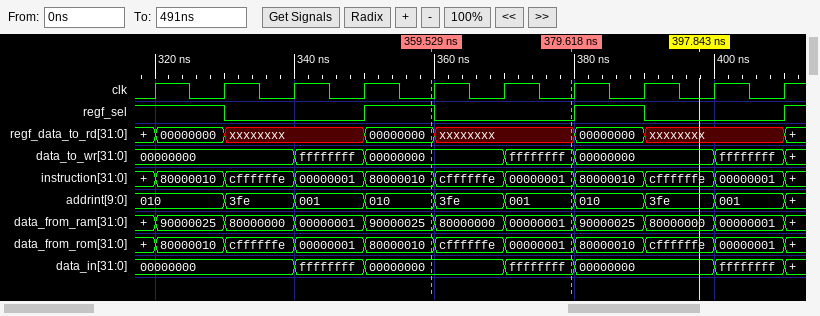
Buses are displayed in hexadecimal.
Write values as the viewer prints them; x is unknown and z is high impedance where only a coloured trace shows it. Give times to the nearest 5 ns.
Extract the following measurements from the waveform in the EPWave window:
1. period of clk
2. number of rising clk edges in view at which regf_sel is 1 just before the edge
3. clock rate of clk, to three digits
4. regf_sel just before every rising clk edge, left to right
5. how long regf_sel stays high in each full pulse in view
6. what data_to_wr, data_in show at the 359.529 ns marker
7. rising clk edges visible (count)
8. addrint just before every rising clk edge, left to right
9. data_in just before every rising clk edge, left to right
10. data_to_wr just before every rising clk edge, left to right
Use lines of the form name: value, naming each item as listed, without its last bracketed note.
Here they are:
period of clk: 10 ns
number of rising clk edges in view at which regf_sel is 1 just before the edge: 4
clock rate of clk, to three digits: 100 MHz
regf_sel just before every rising clk edge, left to right: 1 1 0 0 1 0 0 1 0 0
how long regf_sel stays high in each full pulse in view: 10 ns, 10 ns
what data_to_wr, data_in show at the 359.529 ns marker: data_to_wr=00000000, data_in=00000000
rising clk edges visible: 10
addrint just before every rising clk edge, left to right: 010, 010, 3fe, 001, 010, 3fe, 001, 010, 3fe, 001
data_in just before every rising clk edge, left to right: 00000000, 00000000, 00000000, ffffffff, 00000000, 00000000, ffffffff, 00000000, 00000000, ffffffff
data_to_wr just before every rising clk edge, left to right: 00000000, 00000000, 00000000, ffffffff, 00000000, 00000000, ffffffff, 00000000, 00000000, ffffffff
